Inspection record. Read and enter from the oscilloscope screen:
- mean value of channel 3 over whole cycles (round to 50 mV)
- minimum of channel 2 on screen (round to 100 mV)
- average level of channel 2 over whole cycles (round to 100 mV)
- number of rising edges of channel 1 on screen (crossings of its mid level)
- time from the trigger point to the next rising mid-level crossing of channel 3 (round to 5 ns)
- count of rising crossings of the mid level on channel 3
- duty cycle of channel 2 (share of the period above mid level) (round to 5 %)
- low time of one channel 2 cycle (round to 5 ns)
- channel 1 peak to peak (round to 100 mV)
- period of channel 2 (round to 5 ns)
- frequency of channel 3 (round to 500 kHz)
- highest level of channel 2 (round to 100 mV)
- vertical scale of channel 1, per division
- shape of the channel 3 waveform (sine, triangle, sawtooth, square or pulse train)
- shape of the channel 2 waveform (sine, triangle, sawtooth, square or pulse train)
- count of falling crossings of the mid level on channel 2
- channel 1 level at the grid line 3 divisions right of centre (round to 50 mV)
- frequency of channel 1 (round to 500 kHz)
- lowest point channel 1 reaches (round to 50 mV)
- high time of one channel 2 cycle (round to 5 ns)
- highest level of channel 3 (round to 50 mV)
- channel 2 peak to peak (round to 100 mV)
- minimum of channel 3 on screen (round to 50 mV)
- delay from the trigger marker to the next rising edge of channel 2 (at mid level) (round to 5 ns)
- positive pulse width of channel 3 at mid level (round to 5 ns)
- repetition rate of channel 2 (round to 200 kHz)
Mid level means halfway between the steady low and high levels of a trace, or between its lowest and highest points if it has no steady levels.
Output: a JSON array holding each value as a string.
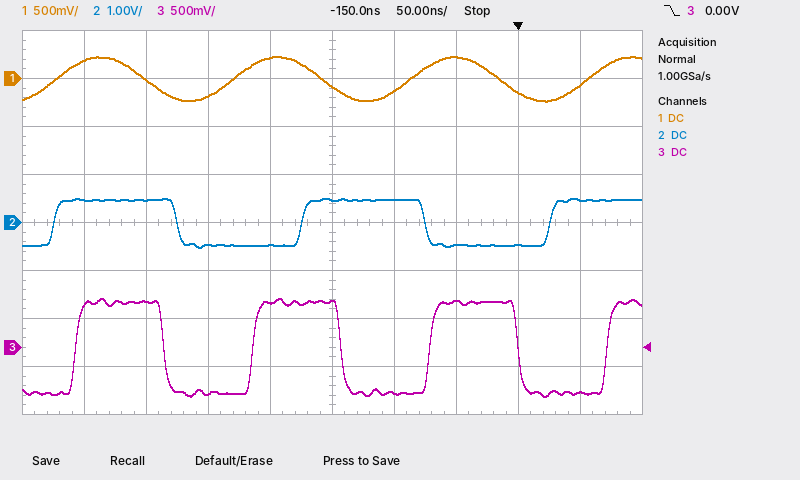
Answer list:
["0 mV", "-500 mV", "0.0 V", "4", "70 ns", "4", "50 %", "100 ns", "500 mV", "200 ns", "7.0 MHz", "500 mV", "500 mV", "square", "square", "2", "-150 mV", "7.0 MHz", "-250 mV", "100 ns", "500 mV", "1.0 V", "-500 mV", "25 ns", "70 ns", "5.0 MHz"]
